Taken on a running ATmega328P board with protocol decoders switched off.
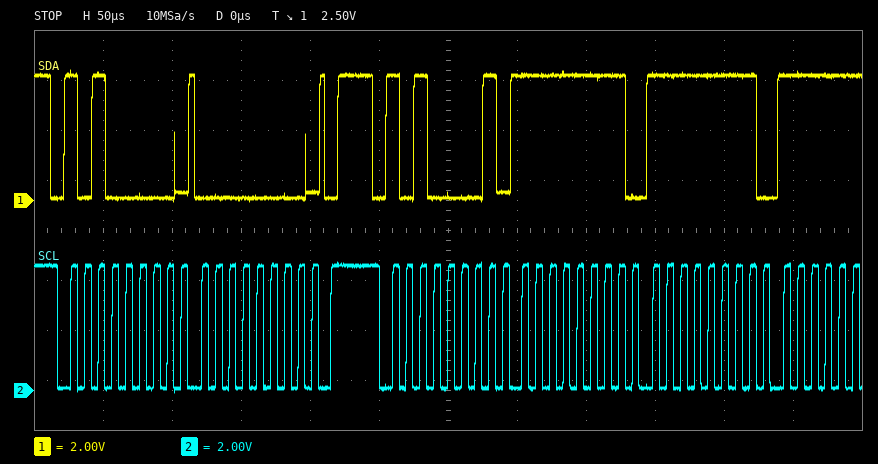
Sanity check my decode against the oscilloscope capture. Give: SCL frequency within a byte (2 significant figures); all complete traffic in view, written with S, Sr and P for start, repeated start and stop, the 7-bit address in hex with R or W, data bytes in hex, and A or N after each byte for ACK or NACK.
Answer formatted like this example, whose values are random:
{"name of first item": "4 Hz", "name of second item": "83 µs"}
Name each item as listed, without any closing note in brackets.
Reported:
{"SCL frequency within a byte": "100 kHz", "all complete traffic in view, written with S, Sr and P for start, repeated start and stop, the 7-bit address in hex with R or W, data bytes in hex, and A or N after each byte for ACK or NACK": "S 50W A 00 A P S 50R A FF A FF A"}
